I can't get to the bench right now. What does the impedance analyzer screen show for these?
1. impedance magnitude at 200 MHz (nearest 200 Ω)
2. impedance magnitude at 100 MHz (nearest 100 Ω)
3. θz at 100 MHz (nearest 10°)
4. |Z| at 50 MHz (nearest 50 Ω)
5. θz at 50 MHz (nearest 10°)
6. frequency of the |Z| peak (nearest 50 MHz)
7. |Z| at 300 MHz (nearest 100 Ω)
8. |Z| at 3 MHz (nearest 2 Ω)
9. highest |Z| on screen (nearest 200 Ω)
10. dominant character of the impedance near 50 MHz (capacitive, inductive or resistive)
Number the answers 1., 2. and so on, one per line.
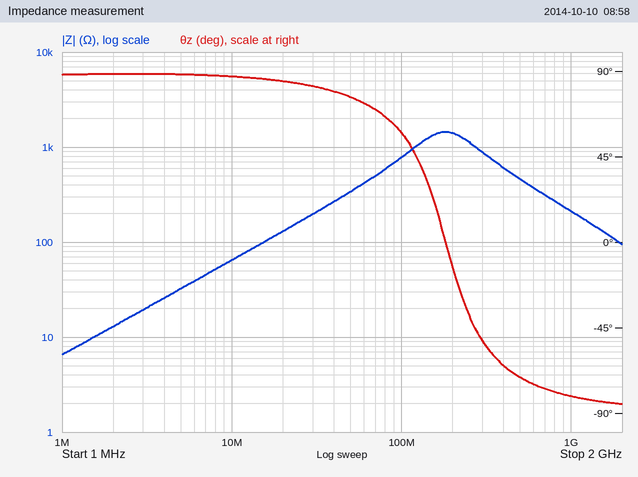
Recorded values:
1. 1.4 kΩ
2. 800 Ω
3. 60°
4. 350 Ω
5. 80°
6. 200 MHz
7. 900 Ω
8. 20 Ω
9. 1.4 kΩ
10. inductive
